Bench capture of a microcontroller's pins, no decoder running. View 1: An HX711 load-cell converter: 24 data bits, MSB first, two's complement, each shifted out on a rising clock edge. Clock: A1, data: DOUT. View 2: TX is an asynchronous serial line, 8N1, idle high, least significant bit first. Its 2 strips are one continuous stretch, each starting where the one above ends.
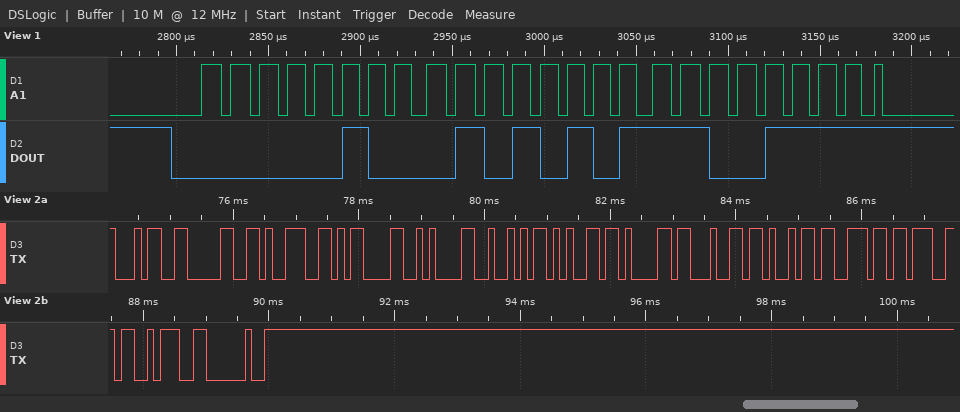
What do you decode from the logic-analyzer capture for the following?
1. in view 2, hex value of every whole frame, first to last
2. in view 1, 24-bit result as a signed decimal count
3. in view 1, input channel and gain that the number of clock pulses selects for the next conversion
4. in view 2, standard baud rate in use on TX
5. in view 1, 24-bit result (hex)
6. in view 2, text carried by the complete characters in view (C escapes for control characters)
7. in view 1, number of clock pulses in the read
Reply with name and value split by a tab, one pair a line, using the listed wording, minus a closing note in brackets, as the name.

in view 2, hex value of every whole frame, first to last	34 30 39 0D 0A 52 65 61 64 69 6E 67 3A 20
in view 1, 24-bit result as a signed decimal count	284111
in view 1, input channel and gain that the number of clock pulses selects for the next conversion	channel A, gain 128
in view 2, standard baud rate in use on TX	9600 baud
in view 1, 24-bit result	0x0455CF
in view 2, text carried by the complete characters in view	"409\r\nReading: "
in view 1, number of clock pulses in the read	25
